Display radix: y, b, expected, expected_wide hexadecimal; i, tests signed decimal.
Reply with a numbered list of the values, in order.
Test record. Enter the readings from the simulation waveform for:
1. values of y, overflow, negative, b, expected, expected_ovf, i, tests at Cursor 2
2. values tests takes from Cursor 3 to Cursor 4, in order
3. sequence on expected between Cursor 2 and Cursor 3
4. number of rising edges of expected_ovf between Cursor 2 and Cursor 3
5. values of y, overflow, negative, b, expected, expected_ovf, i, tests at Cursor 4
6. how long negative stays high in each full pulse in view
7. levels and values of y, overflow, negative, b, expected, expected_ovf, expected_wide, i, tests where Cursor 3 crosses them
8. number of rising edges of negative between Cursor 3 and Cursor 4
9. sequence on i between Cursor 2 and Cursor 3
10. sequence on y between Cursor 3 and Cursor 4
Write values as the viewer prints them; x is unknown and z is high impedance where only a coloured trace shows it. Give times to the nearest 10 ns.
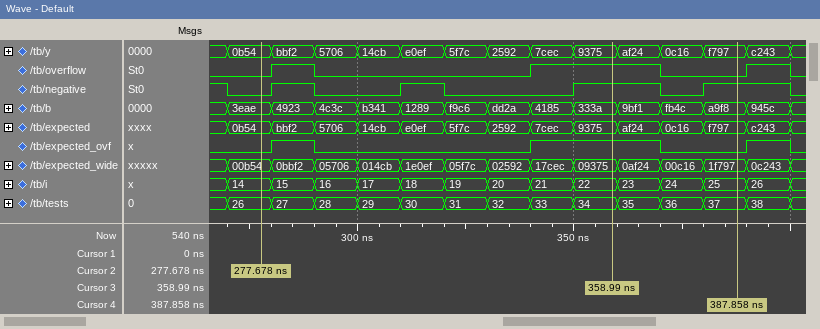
1. y=0b54, overflow=0, negative=0, b=3eae, expected=0b54, expected_ovf=0, i=14, tests=26
2. 34, 35, 36, 37
3. 0b54, bbf2, 5706, 14cb, e0ef, 5f7c, 2592, 7cec, 9375
4. 2
5. y=f797, overflow=0, negative=1, b=a9f8, expected=f797, expected_ovf=0, i=25, tests=37
6. 10 ns, 10 ns, 20 ns, 20 ns
7. y=9375, overflow=1, negative=1, b=333a, expected=9375, expected_ovf=1, expected_wide=09375, i=22, tests=34
8. 1
9. 14, 15, 16, 17, 18, 19, 20, 21, 22
10. 9375, af24, 0c16, f797
